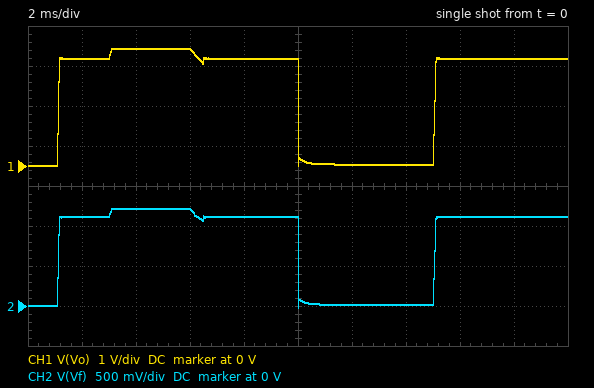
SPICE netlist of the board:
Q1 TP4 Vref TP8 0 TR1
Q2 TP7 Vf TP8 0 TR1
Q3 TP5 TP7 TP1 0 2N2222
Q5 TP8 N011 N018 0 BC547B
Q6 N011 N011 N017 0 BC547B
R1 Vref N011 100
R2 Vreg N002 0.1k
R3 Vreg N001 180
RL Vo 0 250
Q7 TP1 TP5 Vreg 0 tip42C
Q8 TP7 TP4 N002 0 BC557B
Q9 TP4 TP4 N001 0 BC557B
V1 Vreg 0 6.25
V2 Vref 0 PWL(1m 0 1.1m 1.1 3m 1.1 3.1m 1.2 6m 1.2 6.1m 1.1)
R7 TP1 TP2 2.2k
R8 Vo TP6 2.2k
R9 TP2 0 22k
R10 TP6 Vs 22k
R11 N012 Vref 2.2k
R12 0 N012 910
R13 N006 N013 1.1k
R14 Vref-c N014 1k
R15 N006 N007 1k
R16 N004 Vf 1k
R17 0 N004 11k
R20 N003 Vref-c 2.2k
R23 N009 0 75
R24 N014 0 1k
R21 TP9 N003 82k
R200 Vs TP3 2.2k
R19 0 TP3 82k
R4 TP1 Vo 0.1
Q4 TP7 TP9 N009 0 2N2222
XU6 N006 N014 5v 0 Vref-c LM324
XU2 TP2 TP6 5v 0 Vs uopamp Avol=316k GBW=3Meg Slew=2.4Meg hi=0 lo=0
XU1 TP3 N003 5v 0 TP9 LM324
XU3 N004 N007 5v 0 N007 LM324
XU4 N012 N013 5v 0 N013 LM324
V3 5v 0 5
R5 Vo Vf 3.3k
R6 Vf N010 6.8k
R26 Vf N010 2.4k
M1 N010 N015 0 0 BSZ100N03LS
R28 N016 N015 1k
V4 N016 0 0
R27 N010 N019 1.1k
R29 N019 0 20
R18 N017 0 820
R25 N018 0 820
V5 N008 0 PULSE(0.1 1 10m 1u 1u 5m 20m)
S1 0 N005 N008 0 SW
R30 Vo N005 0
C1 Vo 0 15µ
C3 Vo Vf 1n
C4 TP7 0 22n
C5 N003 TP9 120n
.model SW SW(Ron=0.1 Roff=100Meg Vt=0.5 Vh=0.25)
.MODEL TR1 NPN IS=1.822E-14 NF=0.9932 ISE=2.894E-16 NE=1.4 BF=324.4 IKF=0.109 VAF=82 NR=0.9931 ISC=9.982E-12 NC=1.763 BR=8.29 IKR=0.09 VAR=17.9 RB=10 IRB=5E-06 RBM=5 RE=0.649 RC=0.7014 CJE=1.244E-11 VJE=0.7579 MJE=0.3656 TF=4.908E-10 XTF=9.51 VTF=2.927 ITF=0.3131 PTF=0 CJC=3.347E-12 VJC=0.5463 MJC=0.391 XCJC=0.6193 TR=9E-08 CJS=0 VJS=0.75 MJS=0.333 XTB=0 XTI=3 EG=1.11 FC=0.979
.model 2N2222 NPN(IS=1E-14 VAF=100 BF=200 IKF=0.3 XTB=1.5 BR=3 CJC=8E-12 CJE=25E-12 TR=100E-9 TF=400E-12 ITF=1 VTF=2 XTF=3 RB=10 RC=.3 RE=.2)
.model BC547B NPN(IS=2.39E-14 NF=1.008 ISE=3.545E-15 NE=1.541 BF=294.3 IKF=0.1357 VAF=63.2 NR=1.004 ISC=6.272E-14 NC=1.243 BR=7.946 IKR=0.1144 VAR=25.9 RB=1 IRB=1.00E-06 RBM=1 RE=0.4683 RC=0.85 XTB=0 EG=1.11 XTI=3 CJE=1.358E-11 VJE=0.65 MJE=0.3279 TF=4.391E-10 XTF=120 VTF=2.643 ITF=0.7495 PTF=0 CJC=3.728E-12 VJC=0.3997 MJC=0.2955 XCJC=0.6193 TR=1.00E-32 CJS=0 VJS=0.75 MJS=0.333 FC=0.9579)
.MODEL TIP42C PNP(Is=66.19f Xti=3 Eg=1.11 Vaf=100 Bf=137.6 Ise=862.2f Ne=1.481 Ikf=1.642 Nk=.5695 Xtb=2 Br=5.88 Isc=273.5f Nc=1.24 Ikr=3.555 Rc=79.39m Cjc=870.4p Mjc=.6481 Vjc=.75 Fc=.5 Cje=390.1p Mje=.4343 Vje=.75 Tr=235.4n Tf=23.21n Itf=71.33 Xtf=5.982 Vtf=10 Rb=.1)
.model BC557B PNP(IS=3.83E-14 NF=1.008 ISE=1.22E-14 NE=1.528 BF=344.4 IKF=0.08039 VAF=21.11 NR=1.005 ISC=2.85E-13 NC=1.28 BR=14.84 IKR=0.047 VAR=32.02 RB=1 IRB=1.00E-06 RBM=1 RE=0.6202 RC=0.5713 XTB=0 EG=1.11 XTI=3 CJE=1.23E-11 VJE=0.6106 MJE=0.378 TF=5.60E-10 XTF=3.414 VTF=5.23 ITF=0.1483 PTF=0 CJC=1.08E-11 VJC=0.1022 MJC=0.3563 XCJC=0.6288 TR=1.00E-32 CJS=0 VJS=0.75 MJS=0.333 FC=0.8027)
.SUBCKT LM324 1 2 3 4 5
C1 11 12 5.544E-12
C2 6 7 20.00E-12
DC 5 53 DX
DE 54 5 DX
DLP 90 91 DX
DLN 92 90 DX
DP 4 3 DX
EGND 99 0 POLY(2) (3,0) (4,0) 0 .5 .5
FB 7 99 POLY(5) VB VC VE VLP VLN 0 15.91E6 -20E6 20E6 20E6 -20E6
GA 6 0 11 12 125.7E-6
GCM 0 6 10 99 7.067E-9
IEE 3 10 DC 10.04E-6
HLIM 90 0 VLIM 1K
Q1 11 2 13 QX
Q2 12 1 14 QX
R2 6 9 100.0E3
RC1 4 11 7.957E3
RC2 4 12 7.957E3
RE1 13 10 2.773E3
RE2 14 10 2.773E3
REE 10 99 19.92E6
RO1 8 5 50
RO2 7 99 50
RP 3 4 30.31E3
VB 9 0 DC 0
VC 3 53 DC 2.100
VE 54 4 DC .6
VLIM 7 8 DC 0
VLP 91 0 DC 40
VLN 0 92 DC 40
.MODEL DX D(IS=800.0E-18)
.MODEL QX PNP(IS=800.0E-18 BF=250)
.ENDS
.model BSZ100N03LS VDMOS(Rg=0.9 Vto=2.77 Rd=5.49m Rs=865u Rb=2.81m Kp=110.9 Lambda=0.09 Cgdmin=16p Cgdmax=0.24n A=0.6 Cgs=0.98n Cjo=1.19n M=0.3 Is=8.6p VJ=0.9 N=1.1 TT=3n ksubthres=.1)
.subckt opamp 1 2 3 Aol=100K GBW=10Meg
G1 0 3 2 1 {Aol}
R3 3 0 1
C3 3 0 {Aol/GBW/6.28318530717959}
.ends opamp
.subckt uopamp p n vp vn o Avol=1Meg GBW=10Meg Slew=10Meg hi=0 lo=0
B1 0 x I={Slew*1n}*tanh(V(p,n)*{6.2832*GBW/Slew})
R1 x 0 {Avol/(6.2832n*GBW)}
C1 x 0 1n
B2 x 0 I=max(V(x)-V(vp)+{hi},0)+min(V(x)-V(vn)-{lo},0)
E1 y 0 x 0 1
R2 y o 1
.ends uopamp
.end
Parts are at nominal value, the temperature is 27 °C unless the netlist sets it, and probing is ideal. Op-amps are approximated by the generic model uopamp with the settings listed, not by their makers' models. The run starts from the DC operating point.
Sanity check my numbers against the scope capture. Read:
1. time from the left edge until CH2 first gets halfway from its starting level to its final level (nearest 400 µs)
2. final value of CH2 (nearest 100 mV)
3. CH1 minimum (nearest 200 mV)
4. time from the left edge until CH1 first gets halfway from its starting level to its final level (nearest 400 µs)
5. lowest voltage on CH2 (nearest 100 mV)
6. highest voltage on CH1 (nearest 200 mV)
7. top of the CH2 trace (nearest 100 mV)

1.2 ms
1.1 V
0 V
1.2 ms
0 V
3.0 V
1.2 V
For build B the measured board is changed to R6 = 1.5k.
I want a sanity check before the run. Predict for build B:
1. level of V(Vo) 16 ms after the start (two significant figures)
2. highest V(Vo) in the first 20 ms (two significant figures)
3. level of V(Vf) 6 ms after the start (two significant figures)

3.2 V
3.5 V
1.2 V
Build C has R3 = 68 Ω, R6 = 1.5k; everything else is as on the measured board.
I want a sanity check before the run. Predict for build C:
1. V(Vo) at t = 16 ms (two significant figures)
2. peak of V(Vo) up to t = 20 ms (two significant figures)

3.2 V
3.5 V
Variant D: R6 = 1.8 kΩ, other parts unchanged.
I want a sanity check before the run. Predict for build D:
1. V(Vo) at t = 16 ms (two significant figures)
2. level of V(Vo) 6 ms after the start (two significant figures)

3.1 V
3.4 V
